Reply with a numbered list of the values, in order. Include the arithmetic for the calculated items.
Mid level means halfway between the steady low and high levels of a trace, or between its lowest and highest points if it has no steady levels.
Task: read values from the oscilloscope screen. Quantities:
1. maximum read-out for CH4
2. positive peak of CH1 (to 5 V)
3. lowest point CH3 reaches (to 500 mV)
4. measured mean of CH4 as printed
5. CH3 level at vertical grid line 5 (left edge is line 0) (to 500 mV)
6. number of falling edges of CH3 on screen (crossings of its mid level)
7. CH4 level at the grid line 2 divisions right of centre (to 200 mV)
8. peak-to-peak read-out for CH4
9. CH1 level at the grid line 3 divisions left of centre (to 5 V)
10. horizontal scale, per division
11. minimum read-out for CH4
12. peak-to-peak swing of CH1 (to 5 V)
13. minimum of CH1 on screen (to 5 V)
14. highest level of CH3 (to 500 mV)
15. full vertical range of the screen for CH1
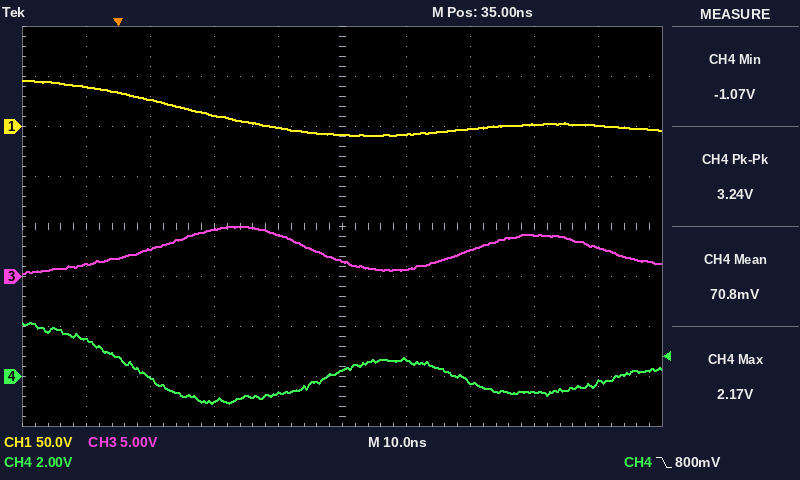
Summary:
1. 2.17 V
2. 45 V
3. 500 mV
4. 70.8 mV
5. 1.5 V
6. 2
7. -200 mV
8. 3.24 V
9. 25 V
10. 10 ns
11. -1.07 V
12. 45 V − (-10 V) = 55 V
13. -10 V
14. 5.0 V
15. 400 V
